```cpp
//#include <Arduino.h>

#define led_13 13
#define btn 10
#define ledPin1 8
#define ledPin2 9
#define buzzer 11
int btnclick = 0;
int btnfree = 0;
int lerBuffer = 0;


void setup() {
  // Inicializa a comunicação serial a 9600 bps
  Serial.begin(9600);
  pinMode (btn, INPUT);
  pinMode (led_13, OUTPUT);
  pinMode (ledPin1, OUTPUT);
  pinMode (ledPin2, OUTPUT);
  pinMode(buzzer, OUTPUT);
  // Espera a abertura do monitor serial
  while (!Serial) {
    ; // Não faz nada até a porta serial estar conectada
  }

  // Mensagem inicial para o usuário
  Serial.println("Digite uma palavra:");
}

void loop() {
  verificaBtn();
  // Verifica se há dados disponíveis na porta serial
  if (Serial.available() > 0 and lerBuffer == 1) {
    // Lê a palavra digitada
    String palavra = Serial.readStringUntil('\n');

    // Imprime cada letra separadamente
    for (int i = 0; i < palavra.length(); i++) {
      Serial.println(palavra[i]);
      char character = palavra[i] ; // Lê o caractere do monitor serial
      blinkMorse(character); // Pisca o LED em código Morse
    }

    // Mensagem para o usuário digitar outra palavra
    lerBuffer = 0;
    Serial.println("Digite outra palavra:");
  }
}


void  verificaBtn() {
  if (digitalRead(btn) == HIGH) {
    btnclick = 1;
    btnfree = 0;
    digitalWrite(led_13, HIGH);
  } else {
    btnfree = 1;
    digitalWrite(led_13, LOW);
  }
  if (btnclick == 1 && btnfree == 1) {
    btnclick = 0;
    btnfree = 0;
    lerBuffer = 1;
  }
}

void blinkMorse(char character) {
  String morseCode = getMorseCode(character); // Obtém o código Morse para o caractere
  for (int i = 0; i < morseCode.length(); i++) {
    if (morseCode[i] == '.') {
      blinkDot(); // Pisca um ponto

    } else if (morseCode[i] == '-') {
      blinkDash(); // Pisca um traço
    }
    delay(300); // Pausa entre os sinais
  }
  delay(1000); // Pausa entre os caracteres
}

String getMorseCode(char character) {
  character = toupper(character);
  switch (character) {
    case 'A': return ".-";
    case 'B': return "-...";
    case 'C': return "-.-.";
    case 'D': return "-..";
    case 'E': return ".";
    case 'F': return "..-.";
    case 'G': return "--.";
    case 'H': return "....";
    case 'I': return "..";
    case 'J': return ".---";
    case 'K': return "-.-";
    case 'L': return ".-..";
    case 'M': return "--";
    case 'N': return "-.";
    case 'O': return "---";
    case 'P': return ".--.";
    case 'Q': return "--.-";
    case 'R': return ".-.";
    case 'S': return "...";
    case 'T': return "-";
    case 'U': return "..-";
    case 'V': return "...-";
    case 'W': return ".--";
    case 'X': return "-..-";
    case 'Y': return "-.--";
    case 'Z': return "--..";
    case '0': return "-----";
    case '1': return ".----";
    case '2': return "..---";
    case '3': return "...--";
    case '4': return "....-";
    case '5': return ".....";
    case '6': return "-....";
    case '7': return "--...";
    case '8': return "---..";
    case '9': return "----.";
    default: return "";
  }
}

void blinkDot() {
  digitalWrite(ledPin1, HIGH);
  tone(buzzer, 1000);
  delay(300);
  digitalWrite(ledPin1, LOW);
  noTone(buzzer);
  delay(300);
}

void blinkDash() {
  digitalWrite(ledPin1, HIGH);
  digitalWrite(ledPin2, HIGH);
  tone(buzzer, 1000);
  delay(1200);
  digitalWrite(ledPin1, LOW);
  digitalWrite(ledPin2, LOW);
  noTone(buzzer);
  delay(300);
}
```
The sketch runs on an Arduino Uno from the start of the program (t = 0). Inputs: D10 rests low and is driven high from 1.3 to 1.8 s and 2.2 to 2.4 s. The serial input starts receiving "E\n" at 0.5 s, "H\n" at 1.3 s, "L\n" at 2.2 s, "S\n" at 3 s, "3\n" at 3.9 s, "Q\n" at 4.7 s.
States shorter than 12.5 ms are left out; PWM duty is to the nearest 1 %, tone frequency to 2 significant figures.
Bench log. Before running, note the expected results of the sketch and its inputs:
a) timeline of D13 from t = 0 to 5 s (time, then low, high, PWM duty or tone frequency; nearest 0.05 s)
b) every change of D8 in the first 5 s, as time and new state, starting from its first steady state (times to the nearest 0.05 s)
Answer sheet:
0 s low; 1.3 s high; 1.8 s low
0 s low; 1.8 s high; 2.1 s low
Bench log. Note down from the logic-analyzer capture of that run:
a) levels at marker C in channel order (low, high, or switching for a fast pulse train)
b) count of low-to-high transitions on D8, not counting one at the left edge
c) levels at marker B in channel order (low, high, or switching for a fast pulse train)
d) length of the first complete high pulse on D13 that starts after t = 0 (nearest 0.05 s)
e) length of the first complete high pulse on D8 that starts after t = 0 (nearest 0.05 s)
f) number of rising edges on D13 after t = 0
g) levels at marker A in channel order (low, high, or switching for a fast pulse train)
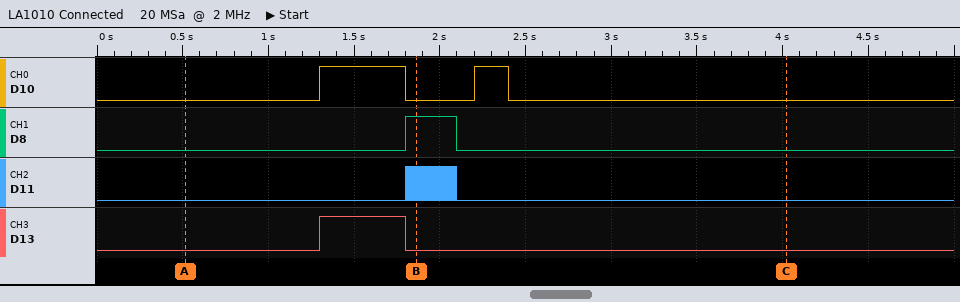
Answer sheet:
D10 low, D8 low, D11 low, D13 low
1
D10 low, D8 high, D11 switching, D13 low
0.50 s
0.30 s
1
D10 low, D8 low, D11 low, D13 low
